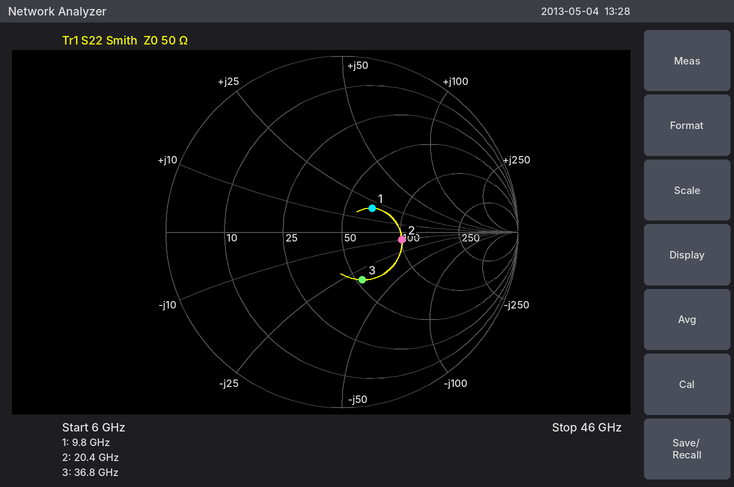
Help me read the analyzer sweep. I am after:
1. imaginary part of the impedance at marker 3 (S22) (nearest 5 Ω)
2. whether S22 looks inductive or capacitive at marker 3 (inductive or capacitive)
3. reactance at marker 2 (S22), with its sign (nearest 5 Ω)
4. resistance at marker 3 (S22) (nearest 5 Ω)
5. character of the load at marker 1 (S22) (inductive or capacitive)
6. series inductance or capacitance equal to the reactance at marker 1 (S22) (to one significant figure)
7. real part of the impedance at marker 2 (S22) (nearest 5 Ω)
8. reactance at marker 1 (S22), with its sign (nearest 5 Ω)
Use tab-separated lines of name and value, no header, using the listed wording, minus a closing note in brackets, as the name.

imaginary part of the impedance at marker 3 (S22)	-30 Ω
whether S22 looks inductive or capacitive at marker 3	capacitive
reactance at marker 2 (S22), with its sign	-10 Ω
resistance at marker 3 (S22)	55 Ω
character of the load at marker 1 (S22)	inductive
series inductance or capacitance equal to the reactance at marker 1 (S22)	300 pH
real part of the impedance at marker 2 (S22)	100 Ω
reactance at marker 1 (S22), with its sign	+20 Ω
